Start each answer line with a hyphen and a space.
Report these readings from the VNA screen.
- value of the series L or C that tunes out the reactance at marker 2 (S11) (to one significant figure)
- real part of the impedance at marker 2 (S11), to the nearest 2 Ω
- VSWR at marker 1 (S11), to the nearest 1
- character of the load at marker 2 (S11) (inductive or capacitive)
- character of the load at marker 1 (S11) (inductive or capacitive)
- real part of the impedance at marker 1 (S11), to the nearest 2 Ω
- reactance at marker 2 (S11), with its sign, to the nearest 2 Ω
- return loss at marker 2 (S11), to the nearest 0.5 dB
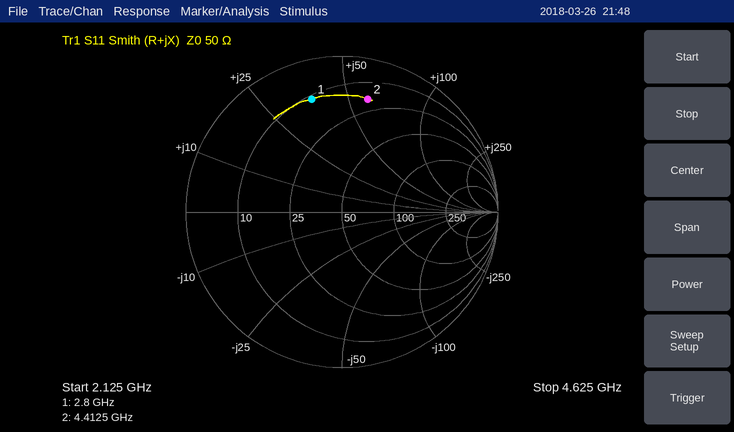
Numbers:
- 600 fF
- 18 Ω
- 7
- inductive
- inductive
- 12 Ω
- +60 Ω
- 2.5 dB
